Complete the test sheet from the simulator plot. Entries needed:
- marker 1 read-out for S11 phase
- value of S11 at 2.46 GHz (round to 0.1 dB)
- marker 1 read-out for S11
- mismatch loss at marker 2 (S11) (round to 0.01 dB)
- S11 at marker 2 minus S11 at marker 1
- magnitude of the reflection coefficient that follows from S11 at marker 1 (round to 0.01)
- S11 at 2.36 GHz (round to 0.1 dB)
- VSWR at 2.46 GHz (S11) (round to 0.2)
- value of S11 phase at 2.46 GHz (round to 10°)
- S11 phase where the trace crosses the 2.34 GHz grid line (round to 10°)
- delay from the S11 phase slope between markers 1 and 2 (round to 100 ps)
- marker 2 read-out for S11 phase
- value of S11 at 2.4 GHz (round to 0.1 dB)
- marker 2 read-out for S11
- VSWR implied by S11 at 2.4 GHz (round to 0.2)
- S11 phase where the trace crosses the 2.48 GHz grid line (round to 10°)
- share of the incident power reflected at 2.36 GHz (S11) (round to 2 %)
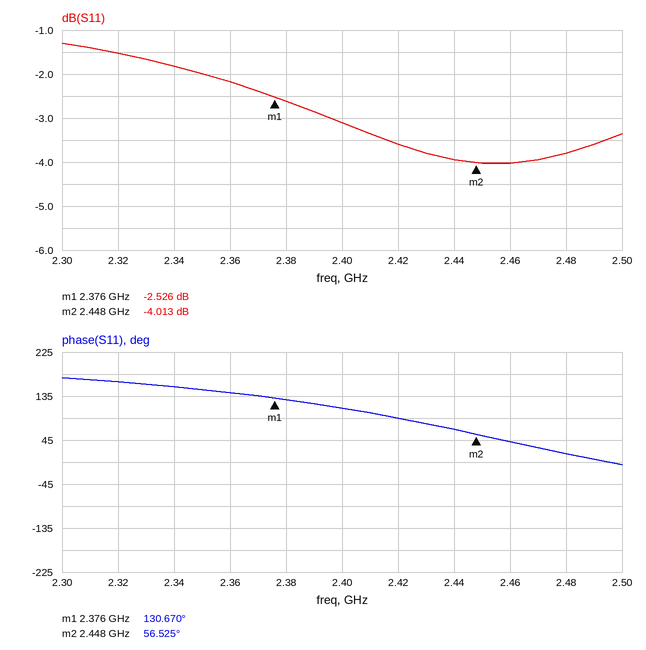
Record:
130.670°
-4.0 dB
-2.526 dB
2.20 dB
-1.487 dB
0.75
-2.2 dB
4.4
40°
150°
2.9 ns
56.525°
-3.1 dB
-4.013 dB
5.6
20°
60 %
